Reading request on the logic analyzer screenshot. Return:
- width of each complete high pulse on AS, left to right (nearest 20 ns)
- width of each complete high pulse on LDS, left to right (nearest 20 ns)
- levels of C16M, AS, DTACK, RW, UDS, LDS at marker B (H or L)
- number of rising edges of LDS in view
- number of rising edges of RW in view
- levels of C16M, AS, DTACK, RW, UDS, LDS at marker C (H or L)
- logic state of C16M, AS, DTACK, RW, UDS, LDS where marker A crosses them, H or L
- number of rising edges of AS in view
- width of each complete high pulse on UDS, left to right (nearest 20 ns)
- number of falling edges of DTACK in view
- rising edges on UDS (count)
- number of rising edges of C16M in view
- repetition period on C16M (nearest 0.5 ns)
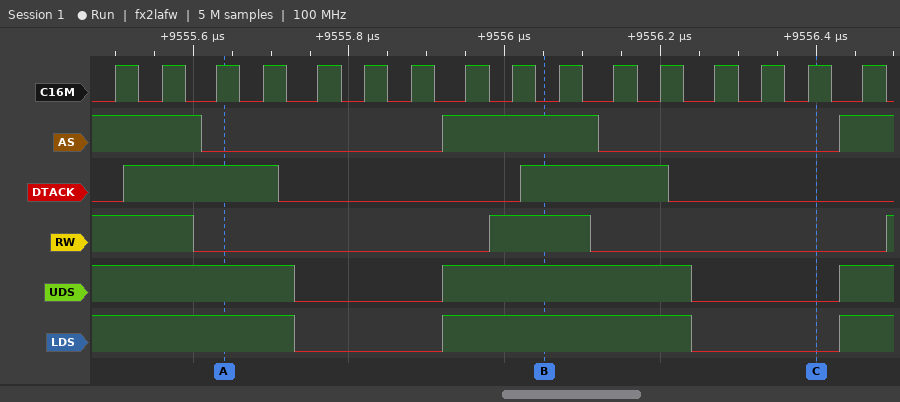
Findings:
200 ns
320 ns
C16M=L, AS=H, DTACK=H, RW=H, UDS=H, LDS=H
2
2
C16M=H, AS=L, DTACK=L, RW=L, UDS=L, LDS=L
C16M=H, AS=L, DTACK=H, RW=L, UDS=H, LDS=H
2
320 ns
2
2
16
64 ns
